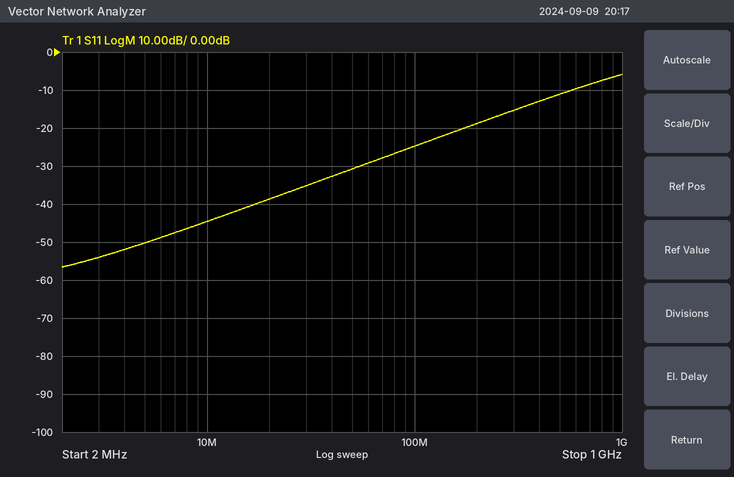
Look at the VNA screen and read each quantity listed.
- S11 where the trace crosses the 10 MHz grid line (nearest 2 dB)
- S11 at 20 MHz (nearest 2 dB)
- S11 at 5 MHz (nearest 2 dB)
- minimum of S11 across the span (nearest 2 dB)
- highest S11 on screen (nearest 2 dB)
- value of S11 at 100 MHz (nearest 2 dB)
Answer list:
-44 dB
-38 dB
-50 dB
-56 dB
-6 dB
-24 dB
